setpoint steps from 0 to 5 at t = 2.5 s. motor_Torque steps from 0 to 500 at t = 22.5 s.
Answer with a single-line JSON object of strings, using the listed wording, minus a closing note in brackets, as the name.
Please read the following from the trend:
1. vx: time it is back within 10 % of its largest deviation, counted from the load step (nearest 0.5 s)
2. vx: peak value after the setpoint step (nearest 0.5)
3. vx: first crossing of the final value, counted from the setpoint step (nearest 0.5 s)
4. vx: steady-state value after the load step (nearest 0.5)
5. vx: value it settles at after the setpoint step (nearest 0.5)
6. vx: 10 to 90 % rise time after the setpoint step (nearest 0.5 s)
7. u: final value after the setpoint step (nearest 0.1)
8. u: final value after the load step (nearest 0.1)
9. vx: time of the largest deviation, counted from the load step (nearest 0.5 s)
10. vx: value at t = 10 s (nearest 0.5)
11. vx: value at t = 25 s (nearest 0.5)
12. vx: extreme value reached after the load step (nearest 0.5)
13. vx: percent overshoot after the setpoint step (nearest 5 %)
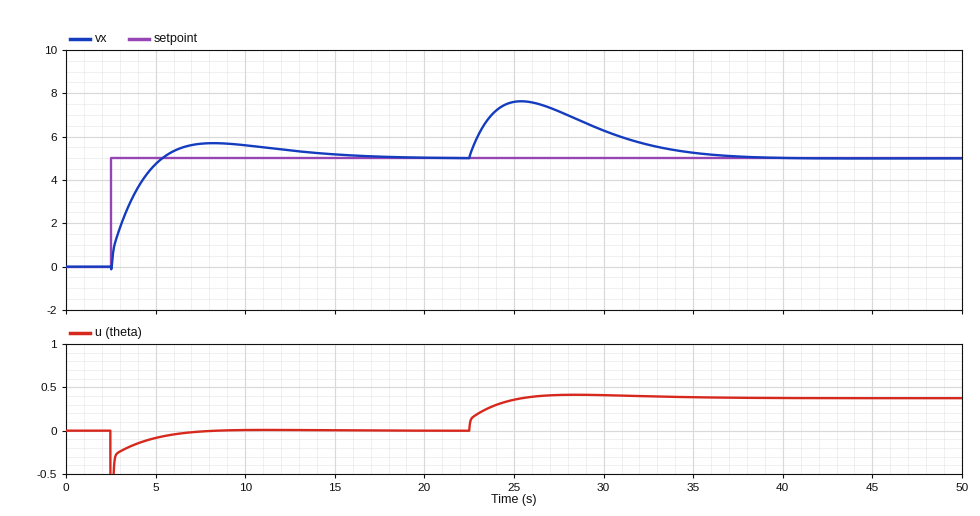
{"vx: time it is back within 10 % of its largest deviation, counted from the load step": "12.5 s", "vx: peak value after the setpoint step": "5.5", "vx: first crossing of the final value, counted from the setpoint step": "3.0 s", "vx: steady-state value after the load step": "5.0", "vx: value it settles at after the setpoint step": "5.0", "vx: 10 to 90 % rise time after the setpoint step": "2.0 s", "u: final value after the setpoint step": "0.0", "u: final value after the load step": "0.4", "vx: time of the largest deviation, counted from the load step": "3.0 s", "vx: value at t = 10 s": "5.5", "vx: value at t = 25 s": "7.5", "vx: extreme value reached after the load step": "7.5", "vx: percent overshoot after the setpoint step": "15 %"}
